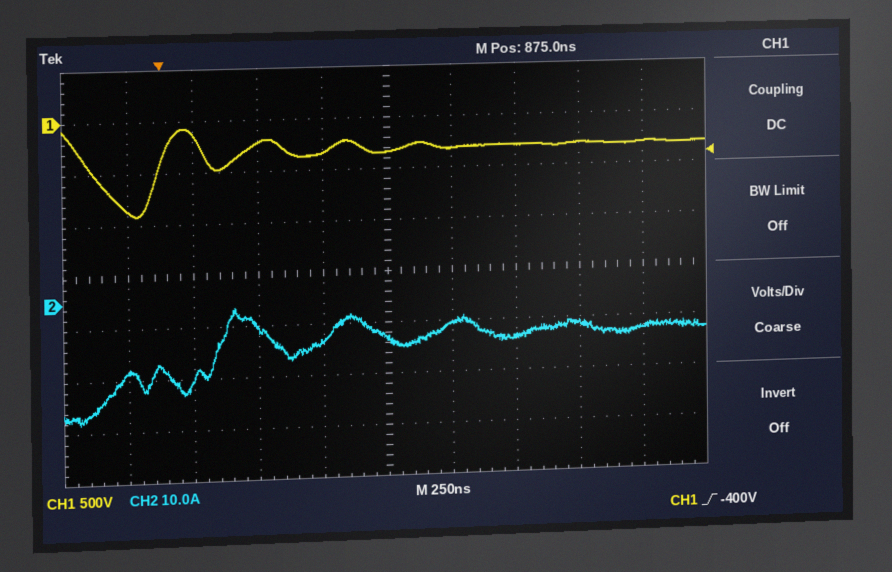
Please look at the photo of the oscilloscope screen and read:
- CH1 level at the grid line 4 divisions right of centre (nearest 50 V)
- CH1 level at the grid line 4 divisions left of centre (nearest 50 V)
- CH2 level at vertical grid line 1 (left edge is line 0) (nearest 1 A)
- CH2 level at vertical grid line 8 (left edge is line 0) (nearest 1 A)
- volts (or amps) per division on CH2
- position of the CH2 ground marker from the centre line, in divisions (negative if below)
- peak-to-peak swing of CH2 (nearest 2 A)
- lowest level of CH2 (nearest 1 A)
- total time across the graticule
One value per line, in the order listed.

-300 V
-850 V
-13 A
-6 A
10 A
-0.5 div
22 A
-23 A
2.5 µs
